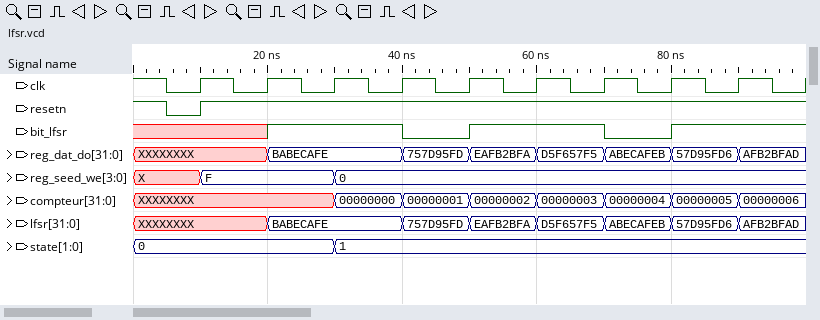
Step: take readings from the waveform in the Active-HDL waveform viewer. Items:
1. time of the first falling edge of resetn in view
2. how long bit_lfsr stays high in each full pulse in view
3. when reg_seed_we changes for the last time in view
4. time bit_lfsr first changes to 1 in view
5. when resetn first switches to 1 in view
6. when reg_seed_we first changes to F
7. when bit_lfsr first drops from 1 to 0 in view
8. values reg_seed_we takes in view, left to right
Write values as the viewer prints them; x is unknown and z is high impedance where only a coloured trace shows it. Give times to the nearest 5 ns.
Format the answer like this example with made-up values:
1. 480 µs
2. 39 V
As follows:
1. 5 ns
2. 20 ns
3. 30 ns
4. 20 ns
5. 10 ns
6. 10 ns
7. 40 ns
8. X, F, 0
